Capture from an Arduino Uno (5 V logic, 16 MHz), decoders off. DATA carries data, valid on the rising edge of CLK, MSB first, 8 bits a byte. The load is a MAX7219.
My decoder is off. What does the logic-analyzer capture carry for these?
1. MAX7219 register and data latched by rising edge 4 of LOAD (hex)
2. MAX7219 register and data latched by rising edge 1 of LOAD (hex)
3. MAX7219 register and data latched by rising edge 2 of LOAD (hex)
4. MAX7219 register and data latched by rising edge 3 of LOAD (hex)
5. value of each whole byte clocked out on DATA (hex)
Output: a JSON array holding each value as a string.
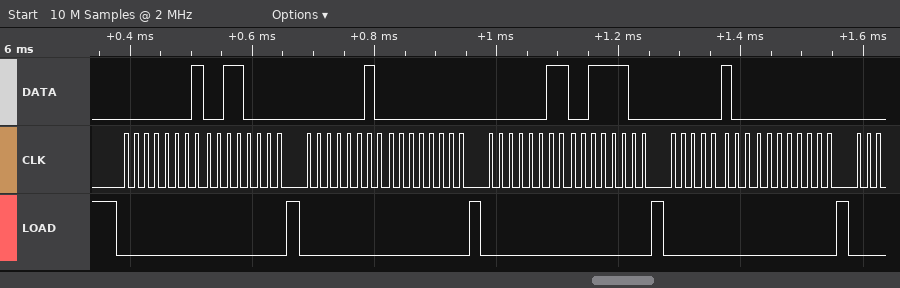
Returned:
["register 0x4, data 0x00", "register 0x1, data 0x30", "register 0x2, data 0x00", "register 0x3, data 0x3C", "01 30 02 00 03 3C 04 00"]
